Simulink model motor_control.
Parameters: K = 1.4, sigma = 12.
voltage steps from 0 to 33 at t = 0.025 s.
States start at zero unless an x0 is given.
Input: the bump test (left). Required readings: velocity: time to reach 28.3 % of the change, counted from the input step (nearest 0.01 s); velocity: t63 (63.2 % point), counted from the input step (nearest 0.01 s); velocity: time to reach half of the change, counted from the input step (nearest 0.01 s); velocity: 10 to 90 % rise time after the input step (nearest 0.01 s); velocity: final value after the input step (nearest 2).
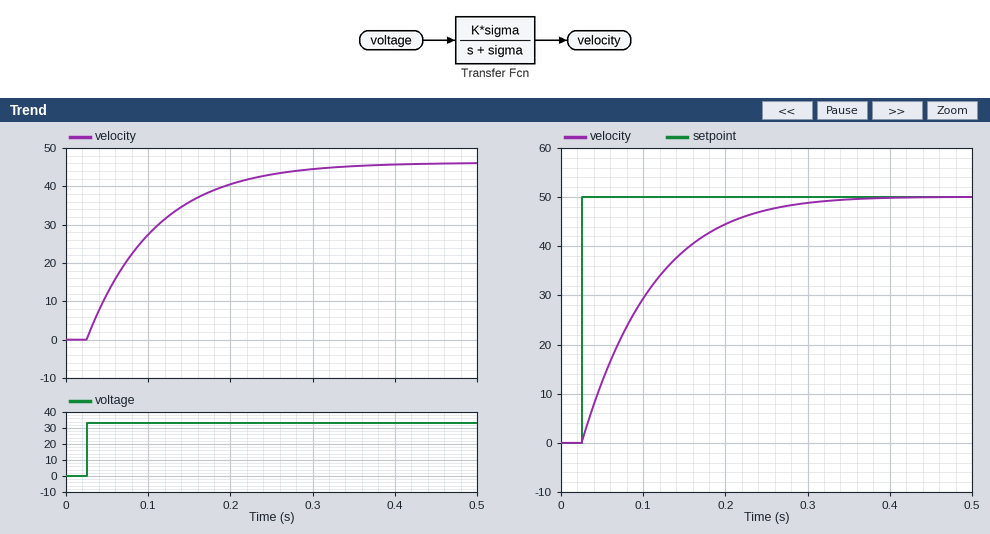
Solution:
0.03 s
0.08 s
0.06 s
0.18 s
46
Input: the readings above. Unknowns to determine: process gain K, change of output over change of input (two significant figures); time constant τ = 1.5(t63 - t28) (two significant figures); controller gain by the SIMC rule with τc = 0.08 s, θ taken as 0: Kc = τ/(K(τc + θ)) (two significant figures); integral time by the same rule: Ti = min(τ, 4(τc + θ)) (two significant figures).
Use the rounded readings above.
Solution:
1.4
0.075 s
0.67
0.075 s
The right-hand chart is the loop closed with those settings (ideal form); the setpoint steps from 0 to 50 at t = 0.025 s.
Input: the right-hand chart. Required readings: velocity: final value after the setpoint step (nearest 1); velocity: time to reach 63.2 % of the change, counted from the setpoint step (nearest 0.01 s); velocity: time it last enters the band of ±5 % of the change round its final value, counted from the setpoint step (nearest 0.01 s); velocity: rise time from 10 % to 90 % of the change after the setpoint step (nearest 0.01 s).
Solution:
50
0.08 s
0.23 s
0.17 s
